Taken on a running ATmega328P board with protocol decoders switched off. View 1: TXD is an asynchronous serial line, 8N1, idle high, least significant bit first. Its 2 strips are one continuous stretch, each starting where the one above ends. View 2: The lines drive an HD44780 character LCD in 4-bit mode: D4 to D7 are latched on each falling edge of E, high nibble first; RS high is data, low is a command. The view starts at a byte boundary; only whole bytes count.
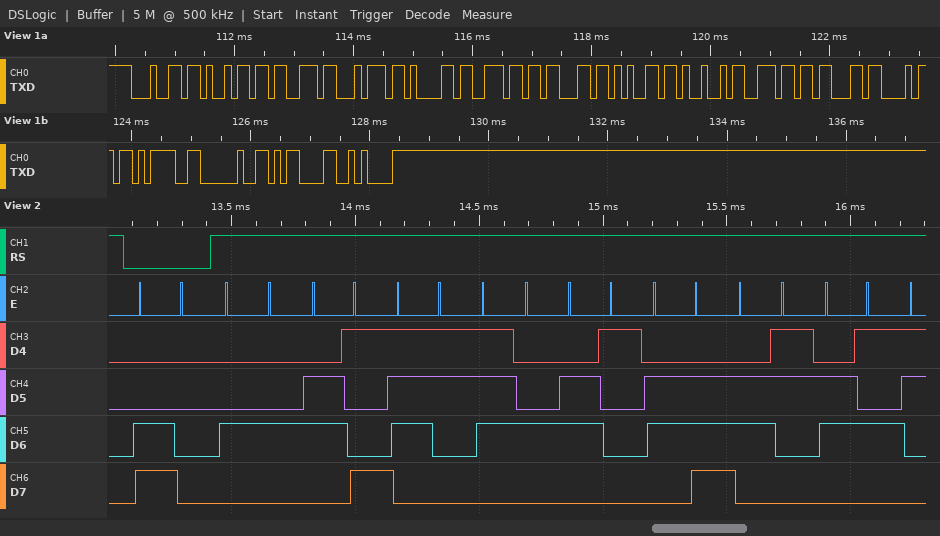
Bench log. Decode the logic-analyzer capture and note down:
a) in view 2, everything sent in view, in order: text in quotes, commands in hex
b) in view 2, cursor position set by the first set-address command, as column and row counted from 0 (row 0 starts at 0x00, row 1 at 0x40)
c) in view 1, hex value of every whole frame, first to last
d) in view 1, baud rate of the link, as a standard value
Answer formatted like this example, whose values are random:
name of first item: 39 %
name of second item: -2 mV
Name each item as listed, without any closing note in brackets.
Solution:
in view 2, everything sent in view, in order: text in quotes, commands in hex: 0xC0 "Distance"
in view 2, cursor position set by the first set-address command, as column and row counted from 0: column 0, row 1
in view 1, hex value of every whole frame, first to last: 0x64 0x69 0x73 0x74 0x61 0x6E 0x63 0x65 0x49 0x6E 0x63 0x68 0x3D 0x20 0x0D 0x0A
in view 1, baud rate of the link, as a standard value: 9600 baud
